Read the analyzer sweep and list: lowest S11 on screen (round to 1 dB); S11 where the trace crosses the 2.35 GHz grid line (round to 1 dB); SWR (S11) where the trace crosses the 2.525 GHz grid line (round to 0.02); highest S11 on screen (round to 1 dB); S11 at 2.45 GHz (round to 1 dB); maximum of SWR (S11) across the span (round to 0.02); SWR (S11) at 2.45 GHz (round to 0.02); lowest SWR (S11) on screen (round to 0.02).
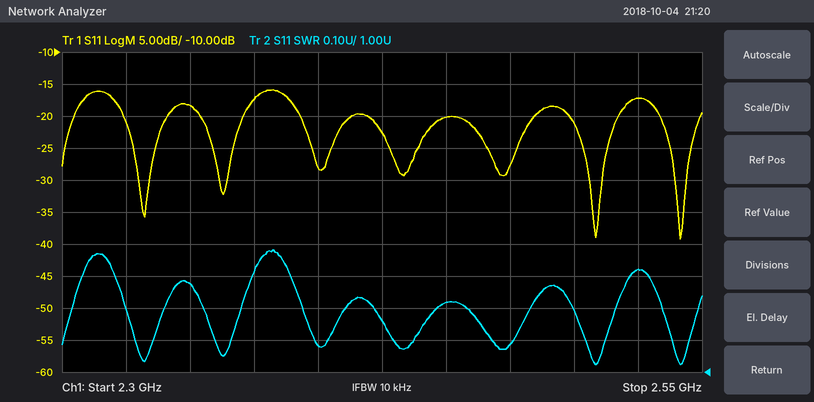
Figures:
-39 dB
-18 dB
1.32
-16 dB
-20 dB
1.38
1.22
1.02
